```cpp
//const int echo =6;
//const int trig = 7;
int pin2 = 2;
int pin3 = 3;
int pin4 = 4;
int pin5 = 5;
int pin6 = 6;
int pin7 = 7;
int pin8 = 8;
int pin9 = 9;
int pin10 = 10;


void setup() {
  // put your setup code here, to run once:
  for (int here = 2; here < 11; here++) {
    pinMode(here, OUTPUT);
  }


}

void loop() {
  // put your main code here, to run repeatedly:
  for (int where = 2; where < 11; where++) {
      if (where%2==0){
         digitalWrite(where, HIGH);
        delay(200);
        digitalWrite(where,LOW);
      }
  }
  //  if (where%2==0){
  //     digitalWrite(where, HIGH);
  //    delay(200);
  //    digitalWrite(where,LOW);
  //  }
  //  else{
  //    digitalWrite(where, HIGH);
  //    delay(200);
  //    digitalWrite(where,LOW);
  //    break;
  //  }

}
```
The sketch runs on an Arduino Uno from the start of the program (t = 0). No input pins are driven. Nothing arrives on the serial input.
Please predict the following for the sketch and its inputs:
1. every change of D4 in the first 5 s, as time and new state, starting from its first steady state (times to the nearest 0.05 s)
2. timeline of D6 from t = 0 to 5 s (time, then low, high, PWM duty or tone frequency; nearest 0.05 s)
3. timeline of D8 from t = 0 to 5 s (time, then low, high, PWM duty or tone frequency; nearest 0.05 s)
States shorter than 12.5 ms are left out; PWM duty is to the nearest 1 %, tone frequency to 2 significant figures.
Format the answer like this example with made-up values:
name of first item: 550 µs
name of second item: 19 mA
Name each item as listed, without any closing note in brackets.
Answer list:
every change of D4 in the first 5 s, as time and new state, starting from its first steady state: 0 s low; 0.2 s high; 0.4 s low; 1.2 s high; 1.4 s low; 2.2 s high; 2.4 s low; 3.2 s high; 3.4 s low; 4.2 s high; 4.4 s low
timeline of D6 from t = 0 to 5 s: 0 s low; 0.4 s high; 0.6 s low; 1.4 s high; 1.6 s low; 2.4 s high; 2.6 s low; 3.4 s high; 3.6 s low; 4.4 s high; 4.6 s low
timeline of D8 from t = 0 to 5 s: 0 s low; 0.6 s high; 0.8 s low; 1.6 s high; 1.8 s low; 2.6 s high; 2.8 s low; 3.6 s high; 3.8 s low; 4.6 s high; 4.8 s low
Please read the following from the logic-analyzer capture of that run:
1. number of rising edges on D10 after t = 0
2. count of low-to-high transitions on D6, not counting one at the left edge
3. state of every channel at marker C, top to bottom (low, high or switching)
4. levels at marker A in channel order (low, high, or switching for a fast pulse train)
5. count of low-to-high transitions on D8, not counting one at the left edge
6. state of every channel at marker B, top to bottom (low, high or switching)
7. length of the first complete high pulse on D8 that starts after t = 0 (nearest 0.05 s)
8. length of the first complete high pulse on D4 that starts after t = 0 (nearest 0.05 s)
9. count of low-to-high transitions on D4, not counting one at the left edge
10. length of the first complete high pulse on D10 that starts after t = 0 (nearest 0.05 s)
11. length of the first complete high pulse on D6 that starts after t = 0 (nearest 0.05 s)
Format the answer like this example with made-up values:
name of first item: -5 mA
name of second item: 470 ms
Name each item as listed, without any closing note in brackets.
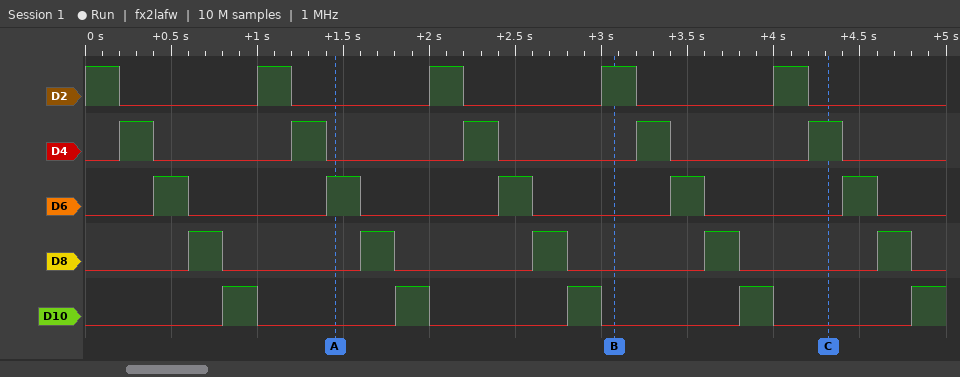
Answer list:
number of rising edges on D10 after t = 0: 5
count of low-to-high transitions on D6, not counting one at the left edge: 5
state of every channel at marker C, top to bottom: D2 low, D4 high, D6 low, D8 low, D10 low
levels at marker A in channel order: D2 low, D4 low, D6 high, D8 low, D10 low
count of low-to-high transitions on D8, not counting one at the left edge: 5
state of every channel at marker B, top to bottom: D2 high, D4 low, D6 low, D8 low, D10 low
length of the first complete high pulse on D8 that starts after t = 0: 0.20 s
length of the first complete high pulse on D4 that starts after t = 0: 0.20 s
count of low-to-high transitions on D4, not counting one at the left edge: 5
length of the first complete high pulse on D10 that starts after t = 0: 0.20 s
length of the first complete high pulse on D6 that starts after t = 0: 0.20 s
